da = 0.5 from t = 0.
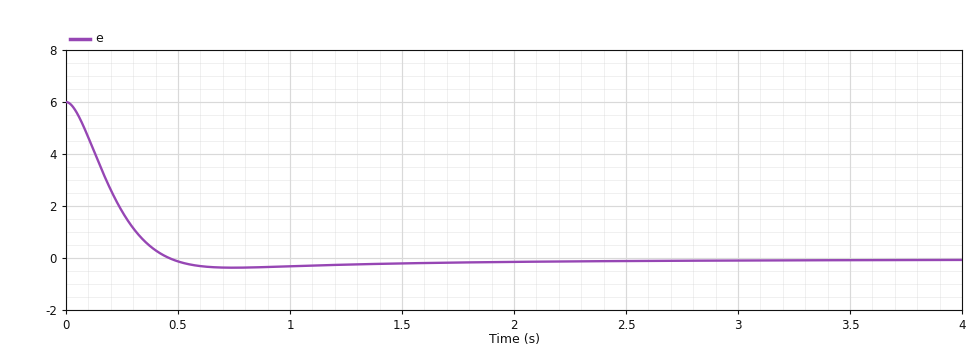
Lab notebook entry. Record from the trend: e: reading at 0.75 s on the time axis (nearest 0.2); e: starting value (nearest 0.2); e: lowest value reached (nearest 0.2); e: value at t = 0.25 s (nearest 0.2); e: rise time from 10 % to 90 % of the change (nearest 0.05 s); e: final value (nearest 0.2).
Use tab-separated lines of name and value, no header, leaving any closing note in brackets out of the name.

e: reading at 0.75 s on the time axis	-0.4
e: starting value	6.0
e: lowest value reached	-0.4
e: value at t = 0.25 s	1.8
e: rise time from 10 % to 90 % of the change	0.30 s
e: final value	0.0
